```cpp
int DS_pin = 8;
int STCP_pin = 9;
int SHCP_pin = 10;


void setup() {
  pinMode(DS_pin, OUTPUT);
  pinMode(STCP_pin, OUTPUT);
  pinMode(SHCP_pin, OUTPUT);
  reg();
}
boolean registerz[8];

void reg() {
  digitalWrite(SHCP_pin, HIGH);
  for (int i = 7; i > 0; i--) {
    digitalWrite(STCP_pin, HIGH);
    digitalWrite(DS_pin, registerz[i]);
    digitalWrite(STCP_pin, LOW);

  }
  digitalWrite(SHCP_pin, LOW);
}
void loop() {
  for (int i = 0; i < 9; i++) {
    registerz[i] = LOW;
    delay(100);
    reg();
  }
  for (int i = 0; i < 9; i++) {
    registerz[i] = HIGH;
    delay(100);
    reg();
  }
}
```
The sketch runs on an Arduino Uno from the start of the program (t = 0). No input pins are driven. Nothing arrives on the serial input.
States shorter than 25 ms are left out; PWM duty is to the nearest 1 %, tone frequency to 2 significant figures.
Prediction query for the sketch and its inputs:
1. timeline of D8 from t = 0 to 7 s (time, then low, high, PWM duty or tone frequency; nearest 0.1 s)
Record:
0 s low; 1.1 s high; 2 s low; 2.9 s high; 3.8 s low; 4.7 s high; 5.6 s low; 6.5 s high
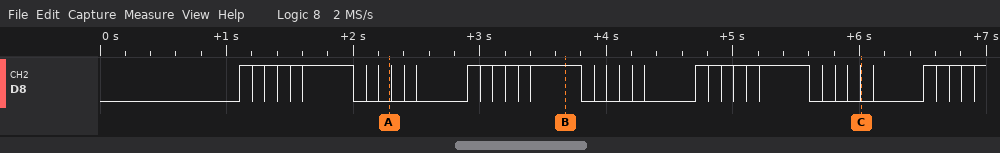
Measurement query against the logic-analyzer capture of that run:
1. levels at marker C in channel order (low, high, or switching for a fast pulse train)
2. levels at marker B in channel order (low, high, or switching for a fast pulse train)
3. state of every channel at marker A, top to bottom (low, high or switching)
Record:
D8 low
D8 high
D8 low
